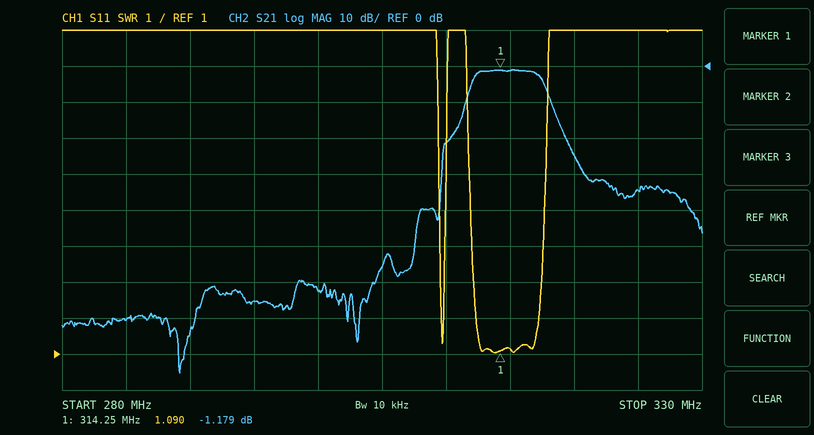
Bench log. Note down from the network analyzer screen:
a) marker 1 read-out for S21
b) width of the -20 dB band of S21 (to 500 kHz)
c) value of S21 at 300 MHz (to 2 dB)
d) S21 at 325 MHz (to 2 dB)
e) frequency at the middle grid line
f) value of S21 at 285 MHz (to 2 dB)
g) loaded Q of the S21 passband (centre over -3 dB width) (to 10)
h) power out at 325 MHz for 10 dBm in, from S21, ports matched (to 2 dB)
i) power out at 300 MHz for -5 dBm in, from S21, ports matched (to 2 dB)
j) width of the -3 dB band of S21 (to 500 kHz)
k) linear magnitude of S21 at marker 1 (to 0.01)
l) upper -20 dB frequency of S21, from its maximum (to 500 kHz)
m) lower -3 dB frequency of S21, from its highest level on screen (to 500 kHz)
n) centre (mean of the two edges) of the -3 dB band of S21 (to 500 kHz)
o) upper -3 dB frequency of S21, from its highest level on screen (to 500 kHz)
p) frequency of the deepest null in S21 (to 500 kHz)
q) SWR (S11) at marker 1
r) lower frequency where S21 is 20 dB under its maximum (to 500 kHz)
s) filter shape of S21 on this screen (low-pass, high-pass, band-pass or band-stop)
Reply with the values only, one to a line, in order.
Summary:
-1.179 dB
9.5 MHz
-62 dB
-34 dB
305 MHz
-70 dB
60
-24 dBm
-68 dBm
5.5 MHz
0.87
319.5 MHz
312.0 MHz
315.0 MHz
317.5 MHz
289.0 MHz
1.090
310.0 MHz
band-pass
